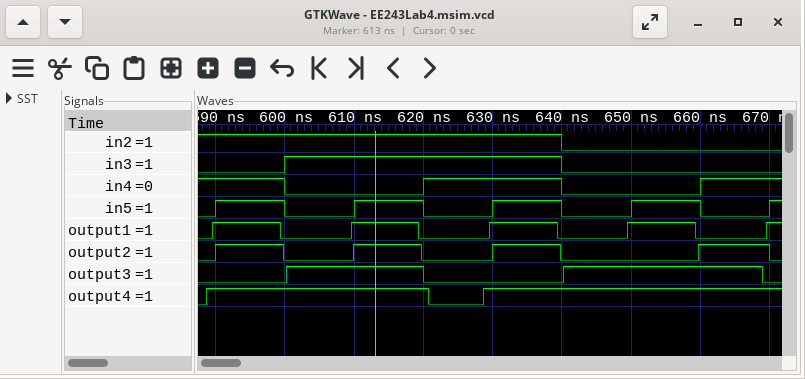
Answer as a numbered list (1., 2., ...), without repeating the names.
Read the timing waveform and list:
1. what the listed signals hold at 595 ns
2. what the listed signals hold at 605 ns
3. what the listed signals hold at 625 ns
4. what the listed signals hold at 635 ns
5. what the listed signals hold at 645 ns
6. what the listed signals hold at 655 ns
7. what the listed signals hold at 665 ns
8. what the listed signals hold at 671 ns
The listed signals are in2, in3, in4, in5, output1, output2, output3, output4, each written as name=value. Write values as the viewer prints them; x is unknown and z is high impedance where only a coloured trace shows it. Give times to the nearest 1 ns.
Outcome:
1. in2=1, in3=0, in4=1, in5=1, output1=1, output2=1, output3=0, output4=1
2. in2=1, in3=1, in4=0, in5=0, output1=0, output2=0, output3=1, output4=1
3. in2=1, in3=1, in4=1, in5=0, output1=0, output2=0, output3=0, output4=0
4. in2=1, in3=1, in4=1, in5=1, output1=1, output2=1, output3=0, output4=1
5. in2=0, in3=0, in4=0, in5=0, output1=0, output2=0, output3=1, output4=1
6. in2=0, in3=0, in4=0, in5=1, output1=1, output2=0, output3=1, output4=1
7. in2=0, in3=0, in4=1, in5=0, output1=0, output2=1, output3=1, output4=1
8. in2=0, in3=0, in4=1, in5=1, output1=1, output2=0, output3=0, output4=1
